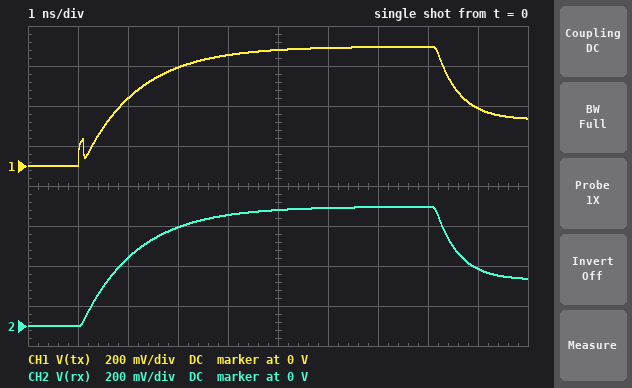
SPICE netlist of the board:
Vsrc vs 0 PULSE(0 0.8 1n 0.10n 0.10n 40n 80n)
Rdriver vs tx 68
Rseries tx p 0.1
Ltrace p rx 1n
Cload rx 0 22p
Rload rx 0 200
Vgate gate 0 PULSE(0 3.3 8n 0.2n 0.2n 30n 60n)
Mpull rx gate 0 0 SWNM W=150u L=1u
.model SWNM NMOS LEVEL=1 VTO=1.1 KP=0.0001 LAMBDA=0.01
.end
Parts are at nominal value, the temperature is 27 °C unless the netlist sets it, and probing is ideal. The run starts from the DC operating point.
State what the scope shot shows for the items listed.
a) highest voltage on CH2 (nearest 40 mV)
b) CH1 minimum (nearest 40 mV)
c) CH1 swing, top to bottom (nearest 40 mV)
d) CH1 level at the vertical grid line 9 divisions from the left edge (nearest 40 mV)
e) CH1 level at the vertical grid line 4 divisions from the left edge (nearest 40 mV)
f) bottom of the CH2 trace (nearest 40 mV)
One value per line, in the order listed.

600 mV
0 V
600 mV
280 mV
560 mV
0 V
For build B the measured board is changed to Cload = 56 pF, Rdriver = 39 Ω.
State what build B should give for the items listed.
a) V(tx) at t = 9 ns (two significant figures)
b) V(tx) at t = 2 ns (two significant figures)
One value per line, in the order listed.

470 mV
260 mV
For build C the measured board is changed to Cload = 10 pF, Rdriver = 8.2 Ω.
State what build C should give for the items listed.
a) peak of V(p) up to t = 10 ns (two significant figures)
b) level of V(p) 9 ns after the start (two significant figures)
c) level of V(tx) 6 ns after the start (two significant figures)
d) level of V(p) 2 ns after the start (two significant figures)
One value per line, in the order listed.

850 mV
630 mV
770 mV
760 mV
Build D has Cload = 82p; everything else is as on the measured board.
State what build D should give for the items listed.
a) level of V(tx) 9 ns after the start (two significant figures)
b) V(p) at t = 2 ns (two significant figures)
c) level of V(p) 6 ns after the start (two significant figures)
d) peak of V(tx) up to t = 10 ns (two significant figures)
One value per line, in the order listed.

390 mV
120 mV
410 mV
490 mV
